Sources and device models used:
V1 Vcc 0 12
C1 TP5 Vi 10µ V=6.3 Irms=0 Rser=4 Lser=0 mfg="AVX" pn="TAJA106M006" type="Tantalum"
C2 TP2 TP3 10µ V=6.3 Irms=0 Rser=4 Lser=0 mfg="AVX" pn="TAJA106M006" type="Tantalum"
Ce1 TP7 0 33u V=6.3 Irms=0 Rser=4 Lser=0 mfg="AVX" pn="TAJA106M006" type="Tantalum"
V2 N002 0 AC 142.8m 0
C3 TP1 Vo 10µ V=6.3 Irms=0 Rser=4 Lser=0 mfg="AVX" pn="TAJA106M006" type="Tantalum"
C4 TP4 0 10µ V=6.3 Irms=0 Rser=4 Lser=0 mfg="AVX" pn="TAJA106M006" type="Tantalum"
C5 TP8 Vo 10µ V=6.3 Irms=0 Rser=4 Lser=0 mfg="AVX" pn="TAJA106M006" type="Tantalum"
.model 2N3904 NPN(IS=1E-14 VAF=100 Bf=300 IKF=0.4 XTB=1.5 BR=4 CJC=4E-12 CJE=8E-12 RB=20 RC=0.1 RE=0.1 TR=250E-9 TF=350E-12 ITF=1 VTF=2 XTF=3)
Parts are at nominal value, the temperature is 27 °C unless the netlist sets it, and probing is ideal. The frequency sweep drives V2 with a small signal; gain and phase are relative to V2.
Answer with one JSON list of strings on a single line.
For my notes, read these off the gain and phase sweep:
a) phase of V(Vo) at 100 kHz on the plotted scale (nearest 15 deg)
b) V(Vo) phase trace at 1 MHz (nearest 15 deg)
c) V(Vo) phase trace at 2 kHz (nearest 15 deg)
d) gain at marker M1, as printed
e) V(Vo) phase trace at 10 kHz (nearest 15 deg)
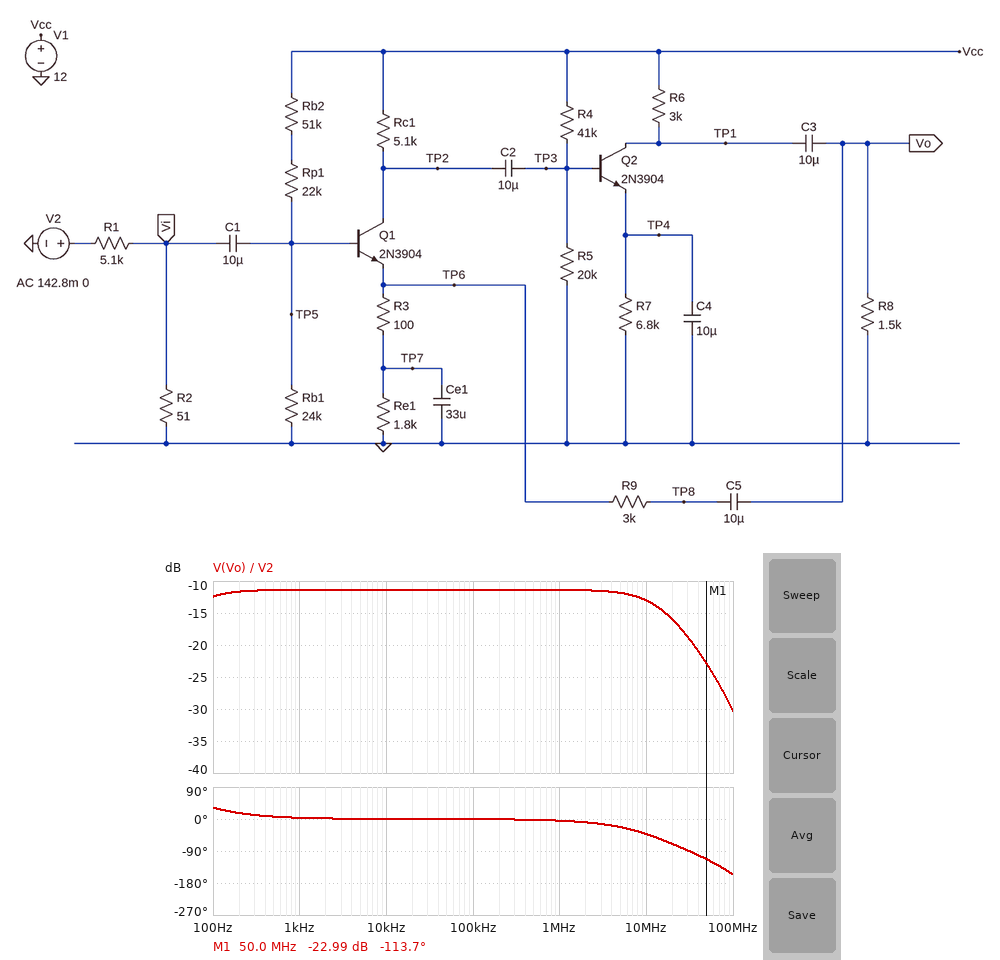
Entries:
["0 deg", "0 deg", "0 deg", "-22.99 dB", "0 deg"]
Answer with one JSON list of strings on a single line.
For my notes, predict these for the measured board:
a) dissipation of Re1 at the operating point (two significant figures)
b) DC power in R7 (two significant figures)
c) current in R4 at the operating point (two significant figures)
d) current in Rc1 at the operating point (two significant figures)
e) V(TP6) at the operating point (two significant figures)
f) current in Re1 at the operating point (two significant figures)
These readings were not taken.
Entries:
["2.5 mW", "1.6 mW", "200 µA", "1.2 mA", "2.2 V", "1.2 mA"]
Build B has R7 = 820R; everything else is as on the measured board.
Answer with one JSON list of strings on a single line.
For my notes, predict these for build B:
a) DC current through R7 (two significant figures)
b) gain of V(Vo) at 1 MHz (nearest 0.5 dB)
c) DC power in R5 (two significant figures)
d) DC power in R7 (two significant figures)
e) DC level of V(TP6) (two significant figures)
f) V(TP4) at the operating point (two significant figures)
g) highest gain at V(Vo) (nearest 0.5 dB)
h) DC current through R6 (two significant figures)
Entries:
["3.2 mA", "-42.0 dB", "540 µW", "8.2 mW", "2.2 V", "2.6 V", "-27.5 dB", "3.1 mA"]
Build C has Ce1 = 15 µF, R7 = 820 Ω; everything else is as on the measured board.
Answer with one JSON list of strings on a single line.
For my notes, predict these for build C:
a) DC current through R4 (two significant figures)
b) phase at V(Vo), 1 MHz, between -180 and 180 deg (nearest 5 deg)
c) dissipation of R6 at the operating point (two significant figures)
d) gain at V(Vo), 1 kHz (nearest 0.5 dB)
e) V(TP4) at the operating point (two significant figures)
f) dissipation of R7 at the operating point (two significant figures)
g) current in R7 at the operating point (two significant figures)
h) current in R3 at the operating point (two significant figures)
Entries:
["210 µA", "-85 deg", "29 mW", "-27.5 dB", "2.6 V", "8.2 mW", "3.2 mA", "1.2 mA"]
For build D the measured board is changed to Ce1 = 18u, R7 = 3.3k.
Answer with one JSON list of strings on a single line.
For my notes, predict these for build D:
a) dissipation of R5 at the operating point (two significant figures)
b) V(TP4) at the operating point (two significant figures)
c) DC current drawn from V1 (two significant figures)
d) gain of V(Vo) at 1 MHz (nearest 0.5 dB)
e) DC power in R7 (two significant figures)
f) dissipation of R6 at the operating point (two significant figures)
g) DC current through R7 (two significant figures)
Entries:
["760 µW", "3.2 V", "2.5 mA", "-11.0 dB", "3.2 mW", "2.9 mW", "980 µA"]
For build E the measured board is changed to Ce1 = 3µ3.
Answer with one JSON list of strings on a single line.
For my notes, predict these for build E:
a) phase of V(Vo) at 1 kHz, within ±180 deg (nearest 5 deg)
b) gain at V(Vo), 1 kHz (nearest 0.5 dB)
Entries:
["25 deg", "-12.5 dB"]
